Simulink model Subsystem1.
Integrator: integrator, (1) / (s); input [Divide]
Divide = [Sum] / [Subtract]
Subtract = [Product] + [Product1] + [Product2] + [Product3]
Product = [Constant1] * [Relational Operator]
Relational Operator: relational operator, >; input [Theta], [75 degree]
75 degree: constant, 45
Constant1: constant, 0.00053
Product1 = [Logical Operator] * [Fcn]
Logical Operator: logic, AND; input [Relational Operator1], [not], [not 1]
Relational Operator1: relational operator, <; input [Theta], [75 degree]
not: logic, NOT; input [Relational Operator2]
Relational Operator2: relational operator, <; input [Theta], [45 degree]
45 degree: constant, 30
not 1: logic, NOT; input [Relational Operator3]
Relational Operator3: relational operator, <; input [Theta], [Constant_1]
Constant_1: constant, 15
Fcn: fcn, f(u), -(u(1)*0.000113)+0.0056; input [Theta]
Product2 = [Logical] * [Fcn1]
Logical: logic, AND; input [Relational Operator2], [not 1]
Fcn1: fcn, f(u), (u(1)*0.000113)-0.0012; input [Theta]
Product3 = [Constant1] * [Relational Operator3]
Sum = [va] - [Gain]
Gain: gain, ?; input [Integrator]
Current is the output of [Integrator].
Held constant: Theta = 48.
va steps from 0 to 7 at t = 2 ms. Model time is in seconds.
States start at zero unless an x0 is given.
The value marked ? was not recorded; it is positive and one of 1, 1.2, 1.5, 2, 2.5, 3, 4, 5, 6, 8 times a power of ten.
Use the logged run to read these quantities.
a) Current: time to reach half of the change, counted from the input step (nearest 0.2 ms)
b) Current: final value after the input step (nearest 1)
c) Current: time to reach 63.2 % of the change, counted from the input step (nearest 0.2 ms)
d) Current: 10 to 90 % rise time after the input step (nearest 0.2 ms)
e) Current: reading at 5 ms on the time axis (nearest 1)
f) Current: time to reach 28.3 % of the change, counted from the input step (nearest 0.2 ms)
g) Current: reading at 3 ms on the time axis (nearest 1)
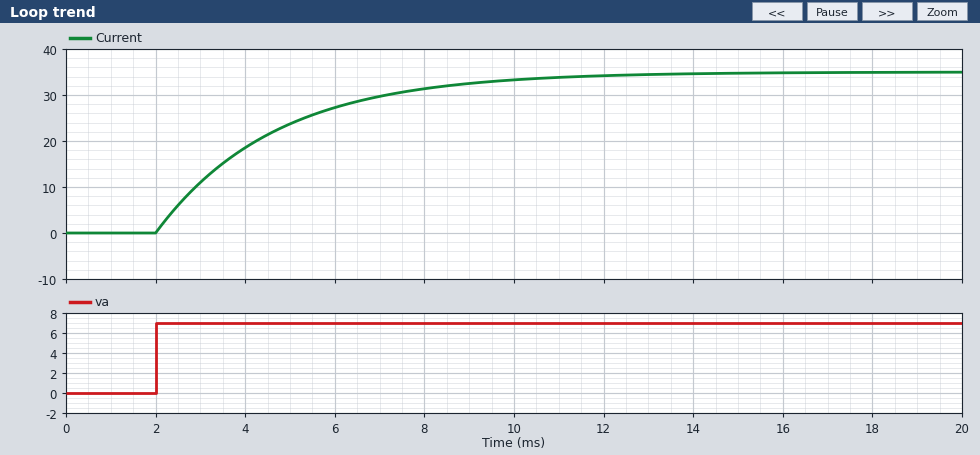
1.8 ms
35
2.6 ms
5.8 ms
24
0.8 ms
11
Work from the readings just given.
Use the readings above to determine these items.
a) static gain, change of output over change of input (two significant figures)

5.0
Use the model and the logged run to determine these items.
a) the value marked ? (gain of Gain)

0.2
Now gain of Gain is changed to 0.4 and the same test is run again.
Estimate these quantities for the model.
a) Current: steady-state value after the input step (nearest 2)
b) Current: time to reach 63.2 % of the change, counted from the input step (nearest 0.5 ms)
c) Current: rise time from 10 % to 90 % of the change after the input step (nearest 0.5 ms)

18
1.5 ms
3.0 ms
